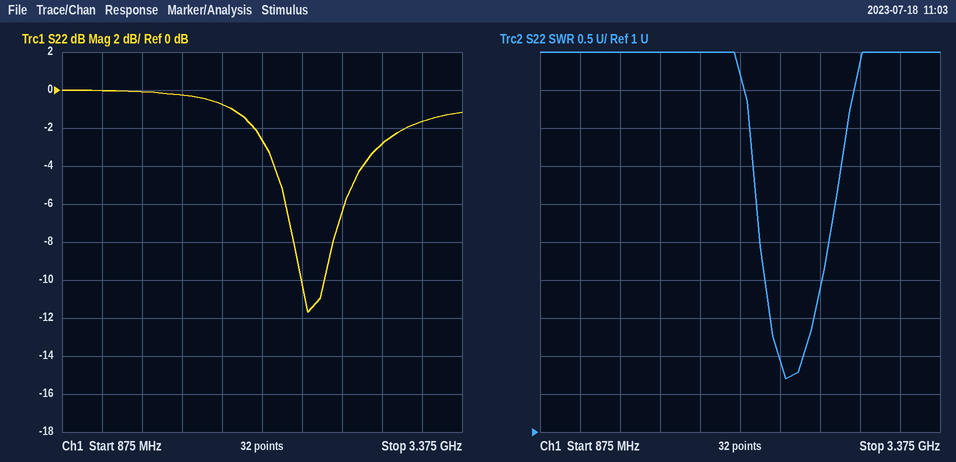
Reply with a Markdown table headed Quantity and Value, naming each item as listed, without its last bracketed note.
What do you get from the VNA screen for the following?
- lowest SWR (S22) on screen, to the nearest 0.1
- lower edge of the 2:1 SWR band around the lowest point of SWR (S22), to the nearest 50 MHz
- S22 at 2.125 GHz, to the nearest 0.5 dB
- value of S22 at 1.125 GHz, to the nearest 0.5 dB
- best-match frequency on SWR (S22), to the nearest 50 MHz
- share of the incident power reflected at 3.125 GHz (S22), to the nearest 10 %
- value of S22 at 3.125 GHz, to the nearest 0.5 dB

| Quantity | Value |
|---|---|
| lowest SWR (S22) on screen, to the nearest 0.1 | 1.7 |
| lower edge of the 2:1 SWR band around the lowest point of SWR (S22), to the nearest 50 MHz | 2.35 GHz |
| S22 at 2.125 GHz, to the nearest 0.5 dB | -2.5 dB |
| value of S22 at 1.125 GHz, to the nearest 0.5 dB | 0.0 dB |
| best-match frequency on SWR (S22), to the nearest 50 MHz | 2.40 GHz |
| share of the incident power reflected at 3.125 GHz (S22), to the nearest 10 % | 70 % |
| value of S22 at 3.125 GHz, to the nearest 0.5 dB | -1.5 dB |
